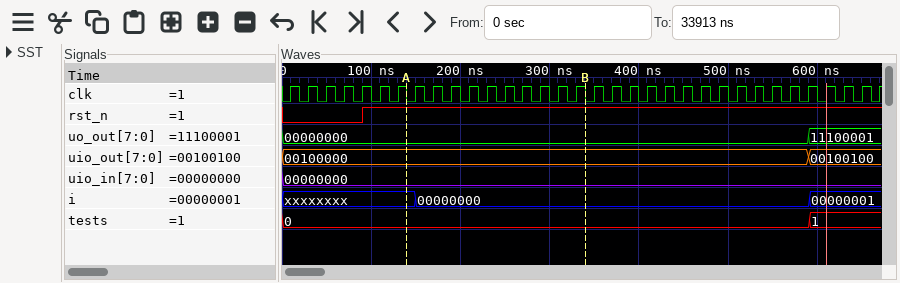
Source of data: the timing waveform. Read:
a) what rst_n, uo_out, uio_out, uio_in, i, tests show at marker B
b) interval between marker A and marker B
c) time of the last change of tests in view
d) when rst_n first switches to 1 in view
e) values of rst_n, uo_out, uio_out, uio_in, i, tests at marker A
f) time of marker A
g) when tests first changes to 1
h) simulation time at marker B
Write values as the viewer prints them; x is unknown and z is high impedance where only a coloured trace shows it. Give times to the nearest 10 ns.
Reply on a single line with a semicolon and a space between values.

rst_n=1, uo_out=00000000, uio_out=00100000, uio_in=00000000, i=00000000, tests=0; 200 ns; 590 ns; 90 ns; rst_n=1, uo_out=00000000, uio_out=00100000, uio_in=00000000, i=xxxxxxxx, tests=0; 140 ns; 590 ns; 340 ns
